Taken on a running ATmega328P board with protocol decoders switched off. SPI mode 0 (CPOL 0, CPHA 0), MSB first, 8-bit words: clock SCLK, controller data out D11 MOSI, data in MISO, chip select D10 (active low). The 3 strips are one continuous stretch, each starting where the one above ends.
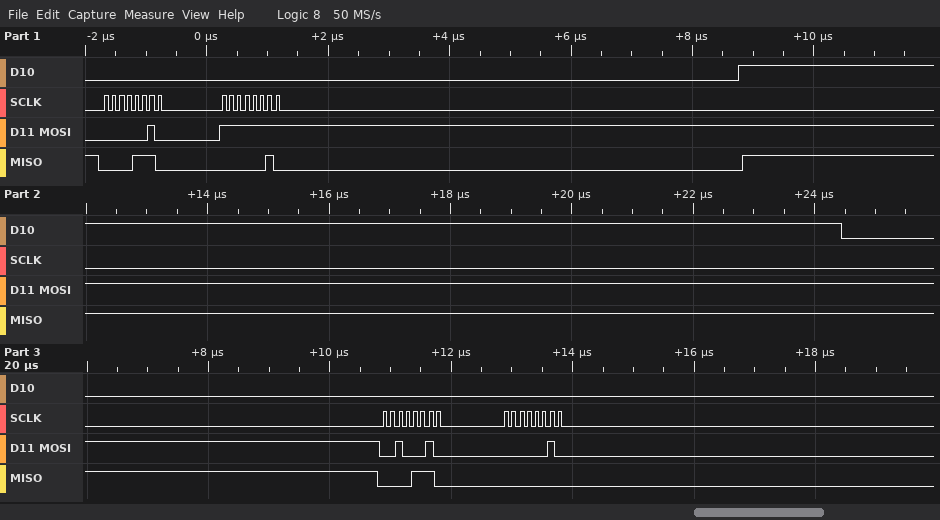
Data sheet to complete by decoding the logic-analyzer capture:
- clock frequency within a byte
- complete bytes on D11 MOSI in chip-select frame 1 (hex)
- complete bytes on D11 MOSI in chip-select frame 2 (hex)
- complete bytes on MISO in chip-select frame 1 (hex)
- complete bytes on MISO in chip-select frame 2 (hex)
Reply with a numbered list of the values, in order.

1. 8 MHz
2. 02 FF
3. 22 02
4. 0E 02
5. 0E 00
